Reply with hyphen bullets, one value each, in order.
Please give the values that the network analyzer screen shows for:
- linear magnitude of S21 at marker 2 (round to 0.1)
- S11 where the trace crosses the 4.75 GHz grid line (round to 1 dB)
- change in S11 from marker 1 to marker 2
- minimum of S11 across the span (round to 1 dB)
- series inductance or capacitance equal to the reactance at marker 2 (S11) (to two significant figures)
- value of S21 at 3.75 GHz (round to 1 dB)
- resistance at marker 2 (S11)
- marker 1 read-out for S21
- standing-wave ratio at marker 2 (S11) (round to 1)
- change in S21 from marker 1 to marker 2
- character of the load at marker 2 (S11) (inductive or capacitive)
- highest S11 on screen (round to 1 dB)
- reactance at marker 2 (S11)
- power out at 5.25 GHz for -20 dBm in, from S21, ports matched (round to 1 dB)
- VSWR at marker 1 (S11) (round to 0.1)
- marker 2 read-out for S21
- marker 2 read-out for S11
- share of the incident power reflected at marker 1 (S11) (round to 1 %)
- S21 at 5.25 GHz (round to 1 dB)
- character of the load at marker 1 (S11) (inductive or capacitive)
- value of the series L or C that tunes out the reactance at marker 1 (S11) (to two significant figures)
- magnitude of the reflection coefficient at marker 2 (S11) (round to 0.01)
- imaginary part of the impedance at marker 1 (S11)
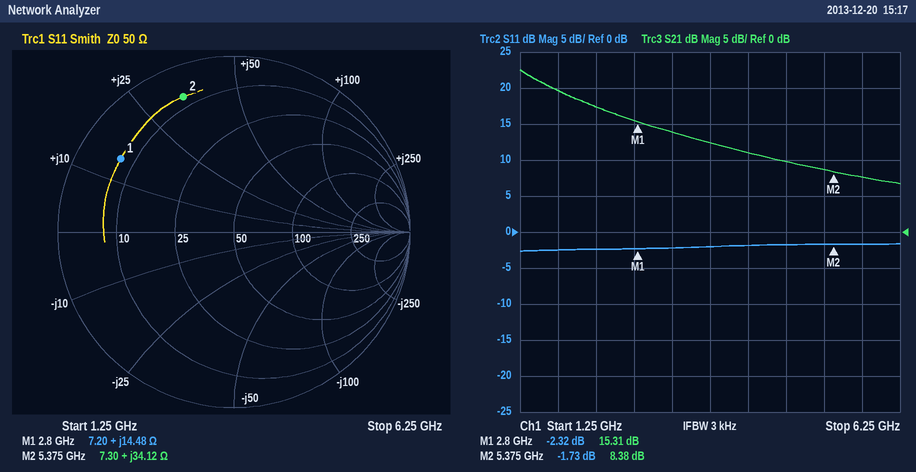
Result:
- 2.6
- -2 dB
- 0.59 dB
- -3 dB
- 1.0 nH
- 12 dB
- 7.30 Ω
- 15.31 dB
- 10
- -6.93 dB
- inductive
- -2 dB
- +34.12 Ω
- -11 dBm
- 7.5
- 8.38 dB
- -1.73 dB
- 59 %
- 9 dB
- inductive
- 3.9 pF
- 0.82
- +14.48 Ω
